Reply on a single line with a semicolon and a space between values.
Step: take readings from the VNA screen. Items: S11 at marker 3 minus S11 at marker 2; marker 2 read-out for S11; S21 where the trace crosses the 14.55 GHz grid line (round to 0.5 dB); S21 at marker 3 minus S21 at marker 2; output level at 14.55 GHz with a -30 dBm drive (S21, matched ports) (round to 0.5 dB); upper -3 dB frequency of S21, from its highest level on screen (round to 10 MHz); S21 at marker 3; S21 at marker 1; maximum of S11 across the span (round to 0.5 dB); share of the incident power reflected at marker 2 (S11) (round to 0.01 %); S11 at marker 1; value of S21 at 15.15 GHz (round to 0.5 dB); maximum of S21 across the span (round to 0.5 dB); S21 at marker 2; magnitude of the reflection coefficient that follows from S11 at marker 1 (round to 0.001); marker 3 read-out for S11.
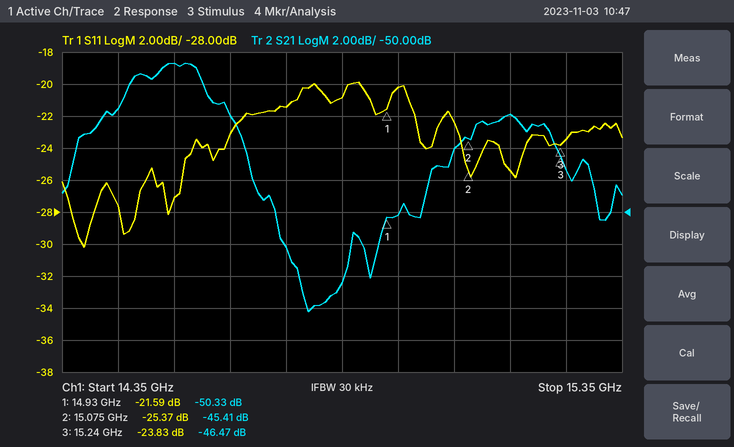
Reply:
1.54 dB; -25.37 dB; -40.5 dB; -1.06 dB; -70.5 dBm; 14.65 GHz; -46.47 dB; -50.33 dB; -20.0 dB; 0.29 %; -21.59 dB; -44.0 dB; -40.5 dB; -45.41 dB; 0.083; -23.83 dB
